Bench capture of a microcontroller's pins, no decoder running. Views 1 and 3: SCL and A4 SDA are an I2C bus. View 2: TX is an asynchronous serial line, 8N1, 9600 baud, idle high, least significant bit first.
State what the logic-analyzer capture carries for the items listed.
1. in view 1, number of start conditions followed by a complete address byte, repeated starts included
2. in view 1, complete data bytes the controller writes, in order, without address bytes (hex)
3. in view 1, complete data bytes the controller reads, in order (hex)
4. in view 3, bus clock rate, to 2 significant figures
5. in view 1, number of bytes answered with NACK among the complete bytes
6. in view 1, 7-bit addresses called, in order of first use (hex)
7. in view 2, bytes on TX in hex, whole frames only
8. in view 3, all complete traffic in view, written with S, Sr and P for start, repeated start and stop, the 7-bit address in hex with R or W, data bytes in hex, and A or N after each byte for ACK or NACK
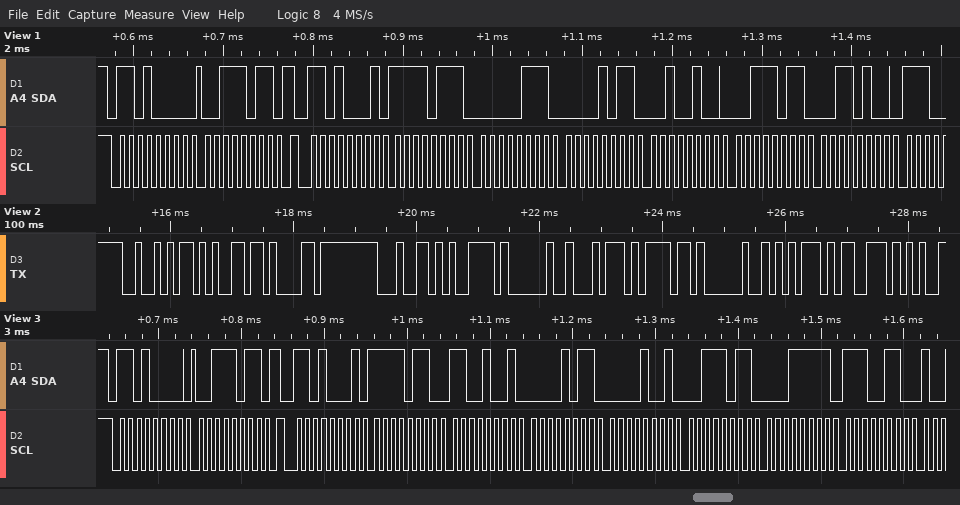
2
3B
F7 07 0B 24 3B 34
100 kHz
0
0x68
52 65 61 64 79 20 74 6F 20 75 73
S 68W A 3B A Sr 68R A F6 A C9 A 0B A 09 A 3B A 1F A E6 A
